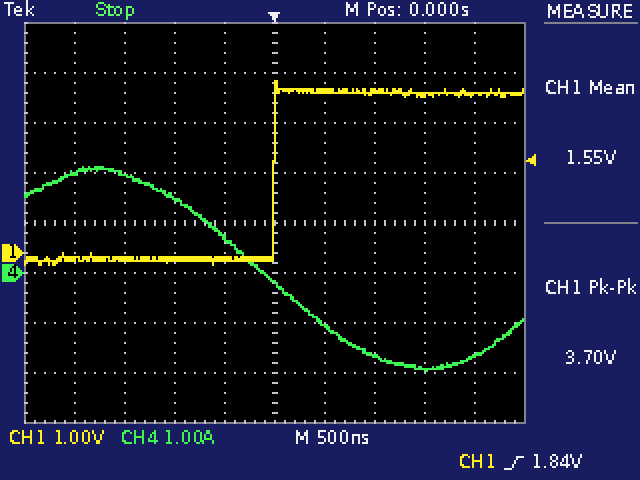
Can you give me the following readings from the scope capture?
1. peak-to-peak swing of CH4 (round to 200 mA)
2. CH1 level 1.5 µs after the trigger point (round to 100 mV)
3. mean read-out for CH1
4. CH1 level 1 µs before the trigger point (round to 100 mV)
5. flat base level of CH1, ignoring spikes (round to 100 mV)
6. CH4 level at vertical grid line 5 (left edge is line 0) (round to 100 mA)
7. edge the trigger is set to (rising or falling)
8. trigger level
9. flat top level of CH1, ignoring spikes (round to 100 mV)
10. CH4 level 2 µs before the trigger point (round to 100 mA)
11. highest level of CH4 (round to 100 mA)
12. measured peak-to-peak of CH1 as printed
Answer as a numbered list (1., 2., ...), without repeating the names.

1. 4.0 A
2. 3.2 V
3. 1.55 V
4. -100 mV
5. -100 mV
6. -200 mA
7. rising
8. 1.84 V
9. 3.2 V
10. 2.0 A
11. 2.1 A
12. 3.70 V
